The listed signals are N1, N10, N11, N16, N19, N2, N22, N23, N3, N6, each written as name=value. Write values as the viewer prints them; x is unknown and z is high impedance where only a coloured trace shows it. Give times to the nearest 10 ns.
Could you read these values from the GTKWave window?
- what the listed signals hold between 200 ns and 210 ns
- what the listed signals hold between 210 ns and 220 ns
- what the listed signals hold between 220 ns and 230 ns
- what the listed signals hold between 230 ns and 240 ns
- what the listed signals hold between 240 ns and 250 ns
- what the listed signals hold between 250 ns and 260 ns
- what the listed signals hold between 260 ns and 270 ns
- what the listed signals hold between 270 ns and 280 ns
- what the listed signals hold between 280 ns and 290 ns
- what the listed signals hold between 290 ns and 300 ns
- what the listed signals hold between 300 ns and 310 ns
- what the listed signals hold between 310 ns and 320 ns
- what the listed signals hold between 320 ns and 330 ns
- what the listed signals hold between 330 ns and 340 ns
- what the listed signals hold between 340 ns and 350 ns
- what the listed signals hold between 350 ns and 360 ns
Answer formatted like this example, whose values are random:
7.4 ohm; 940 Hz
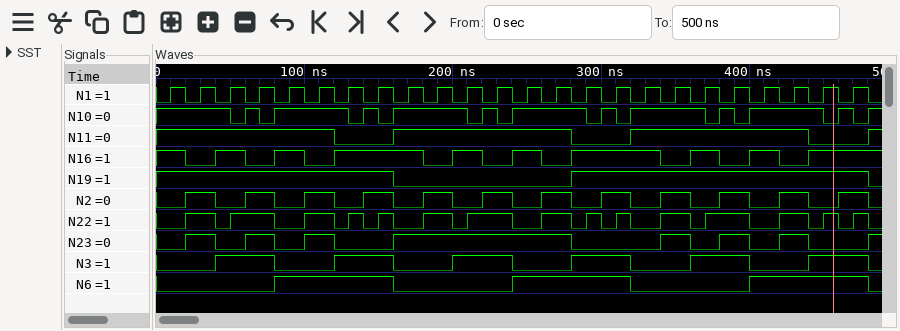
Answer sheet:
N1=0, N10=1, N11=1, N16=1, N19=0, N2=0, N22=0, N23=1, N3=1, N6=0; N1=1, N10=0, N11=1, N16=1, N19=0, N2=0, N22=1, N23=1, N3=1, N6=0; N1=0, N10=1, N11=1, N16=0, N19=0, N2=1, N22=1, N23=1, N3=1, N6=0; N1=1, N10=0, N11=1, N16=0, N19=0, N2=1, N22=1, N23=1, N3=1, N6=0; N1=0, N10=1, N11=1, N16=1, N19=0, N2=0, N22=0, N23=1, N3=0, N6=1; N1=1, N10=1, N11=1, N16=1, N19=0, N2=0, N22=0, N23=1, N3=0, N6=1; N1=0, N10=1, N11=1, N16=0, N19=0, N2=1, N22=1, N23=1, N3=0, N6=1; N1=1, N10=1, N11=1, N16=0, N19=0, N2=1, N22=1, N23=1, N3=0, N6=1; N1=0, N10=1, N11=0, N16=1, N19=1, N2=0, N22=0, N23=0, N3=1, N6=1; N1=1, N10=0, N11=0, N16=1, N19=1, N2=0, N22=1, N23=0, N3=1, N6=1; N1=0, N10=1, N11=0, N16=1, N19=1, N2=1, N22=0, N23=0, N3=1, N6=1; N1=1, N10=0, N11=0, N16=1, N19=1, N2=1, N22=1, N23=0, N3=1, N6=1; N1=0, N10=1, N11=1, N16=1, N19=1, N2=0, N22=0, N23=0, N3=0, N6=0; N1=1, N10=1, N11=1, N16=1, N19=1, N2=0, N22=0, N23=0, N3=0, N6=0; N1=0, N10=1, N11=1, N16=0, N19=1, N2=1, N22=1, N23=1, N3=0, N6=0; N1=1, N10=1, N11=1, N16=0, N19=1, N2=1, N22=1, N23=1, N3=0, N6=0
